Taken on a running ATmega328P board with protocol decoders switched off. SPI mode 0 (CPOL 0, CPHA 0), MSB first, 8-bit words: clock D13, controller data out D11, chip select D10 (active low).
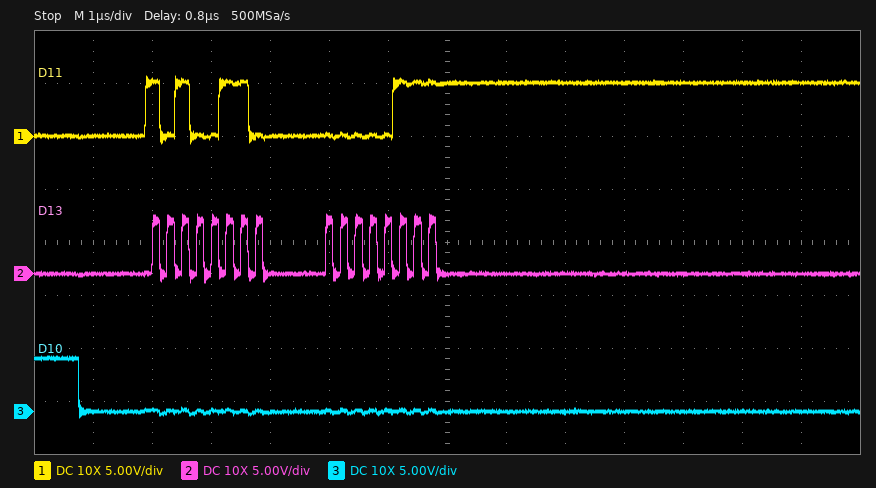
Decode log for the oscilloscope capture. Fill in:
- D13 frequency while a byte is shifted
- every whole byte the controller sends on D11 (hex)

4 MHz
A6 07
